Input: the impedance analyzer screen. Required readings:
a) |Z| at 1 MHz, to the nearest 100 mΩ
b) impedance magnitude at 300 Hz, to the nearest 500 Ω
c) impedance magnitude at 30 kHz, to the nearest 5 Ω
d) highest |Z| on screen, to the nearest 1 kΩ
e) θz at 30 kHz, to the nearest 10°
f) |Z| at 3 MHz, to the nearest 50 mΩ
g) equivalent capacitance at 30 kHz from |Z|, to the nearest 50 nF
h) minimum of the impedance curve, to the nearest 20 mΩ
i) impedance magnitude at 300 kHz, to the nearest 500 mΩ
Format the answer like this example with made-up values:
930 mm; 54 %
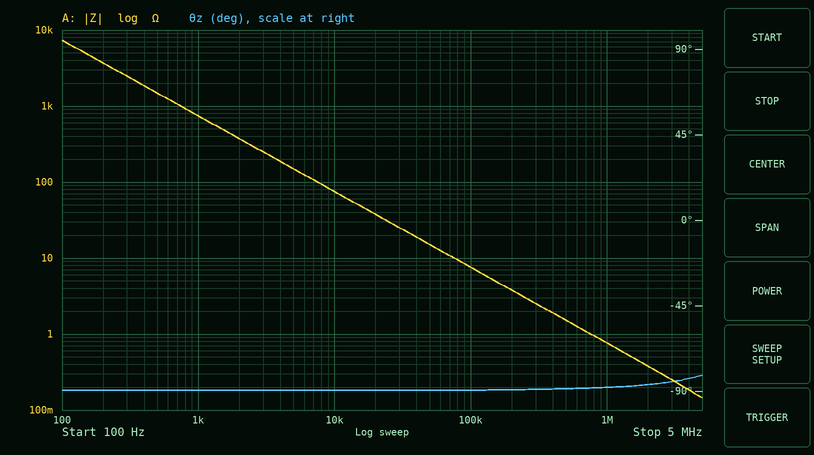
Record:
800 mΩ; 2.5 kΩ; 25 Ω; 7 kΩ; -90°; 250 mΩ; 200 nF; 140 mΩ; 2.5 Ω
